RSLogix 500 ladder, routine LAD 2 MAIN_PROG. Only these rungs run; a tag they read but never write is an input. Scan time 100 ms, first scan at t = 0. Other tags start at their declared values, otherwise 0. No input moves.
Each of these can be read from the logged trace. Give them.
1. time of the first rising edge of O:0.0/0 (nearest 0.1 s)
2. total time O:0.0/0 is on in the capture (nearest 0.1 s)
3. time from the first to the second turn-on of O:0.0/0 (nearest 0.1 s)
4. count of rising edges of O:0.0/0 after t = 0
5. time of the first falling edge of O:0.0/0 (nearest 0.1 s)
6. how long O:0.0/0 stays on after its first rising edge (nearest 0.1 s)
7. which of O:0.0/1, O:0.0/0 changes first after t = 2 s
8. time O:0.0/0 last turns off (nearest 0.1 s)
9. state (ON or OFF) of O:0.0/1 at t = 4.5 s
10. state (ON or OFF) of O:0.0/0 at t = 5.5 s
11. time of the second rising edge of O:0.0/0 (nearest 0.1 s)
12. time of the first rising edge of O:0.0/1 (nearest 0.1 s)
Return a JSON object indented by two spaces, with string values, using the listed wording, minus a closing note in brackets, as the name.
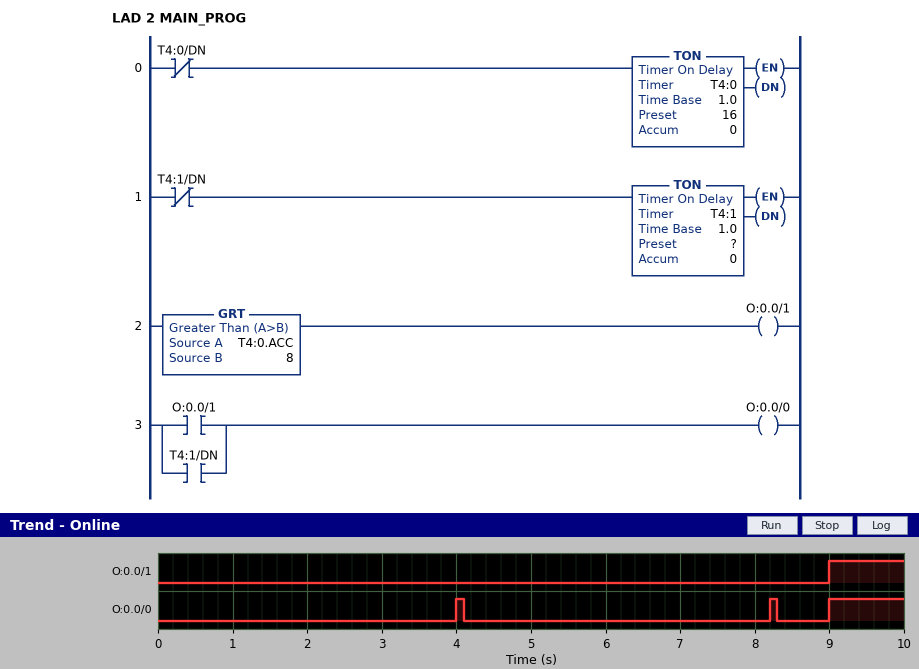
{
  "time of the first rising edge of O:0.0/0": "4.0 s",
  "total time O:0.0/0 is on in the capture": "1.2 s",
  "time from the first to the second turn-on of O:0.0/0": "4.2 s",
  "count of rising edges of O:0.0/0 after t = 0": "3",
  "time of the first falling edge of O:0.0/0": "4.1 s",
  "how long O:0.0/0 stays on after its first rising edge": "0.1 s",
  "which of O:0.0/1, O:0.0/0 changes first after t = 2 s": "O:0.0/0",
  "time O:0.0/0 last turns off": "8.3 s",
  "state (ON or OFF) of O:0.0/1 at t = 4.5 s": "OFF",
  "state (ON or OFF) of O:0.0/0 at t = 5.5 s": "OFF",
  "time of the second rising edge of O:0.0/0": "8.2 s",
  "time of the first rising edge of O:0.0/1": "9.0 s"
}
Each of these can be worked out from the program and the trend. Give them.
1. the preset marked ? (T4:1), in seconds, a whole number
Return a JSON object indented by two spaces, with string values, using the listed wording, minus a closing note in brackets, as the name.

{
  "the preset marked ? (T4:1), in seconds, a whole number": "4 s"
}
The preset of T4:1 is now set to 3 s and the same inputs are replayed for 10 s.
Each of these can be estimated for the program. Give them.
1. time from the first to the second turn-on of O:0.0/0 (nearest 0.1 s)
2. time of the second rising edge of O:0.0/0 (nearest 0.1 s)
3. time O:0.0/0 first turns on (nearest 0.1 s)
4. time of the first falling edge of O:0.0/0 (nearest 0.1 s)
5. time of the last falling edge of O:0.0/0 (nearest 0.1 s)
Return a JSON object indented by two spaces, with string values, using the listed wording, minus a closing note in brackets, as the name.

{
  "time from the first to the second turn-on of O:0.0/0": "3.2 s",
  "time of the second rising edge of O:0.0/0": "6.2 s",
  "time O:0.0/0 first turns on": "3.0 s",
  "time of the first falling edge of O:0.0/0": "3.1 s",
  "time of the last falling edge of O:0.0/0": "6.3 s"
}
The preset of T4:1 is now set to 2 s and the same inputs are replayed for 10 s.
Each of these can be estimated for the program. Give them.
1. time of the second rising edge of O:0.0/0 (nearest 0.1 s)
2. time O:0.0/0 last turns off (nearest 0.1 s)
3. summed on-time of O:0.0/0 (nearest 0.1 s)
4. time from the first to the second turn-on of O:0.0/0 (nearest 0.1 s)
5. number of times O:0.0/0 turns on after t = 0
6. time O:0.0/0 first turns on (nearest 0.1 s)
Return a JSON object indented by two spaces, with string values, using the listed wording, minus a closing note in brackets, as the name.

{
  "time of the second rising edge of O:0.0/0": "4.2 s",
  "time O:0.0/0 last turns off": "8.7 s",
  "summed on-time of O:0.0/0": "1.4 s",
  "time from the first to the second turn-on of O:0.0/0": "2.2 s",
  "number of times O:0.0/0 turns on after t = 0": "5",
  "time O:0.0/0 first turns on": "2.0 s"
}
